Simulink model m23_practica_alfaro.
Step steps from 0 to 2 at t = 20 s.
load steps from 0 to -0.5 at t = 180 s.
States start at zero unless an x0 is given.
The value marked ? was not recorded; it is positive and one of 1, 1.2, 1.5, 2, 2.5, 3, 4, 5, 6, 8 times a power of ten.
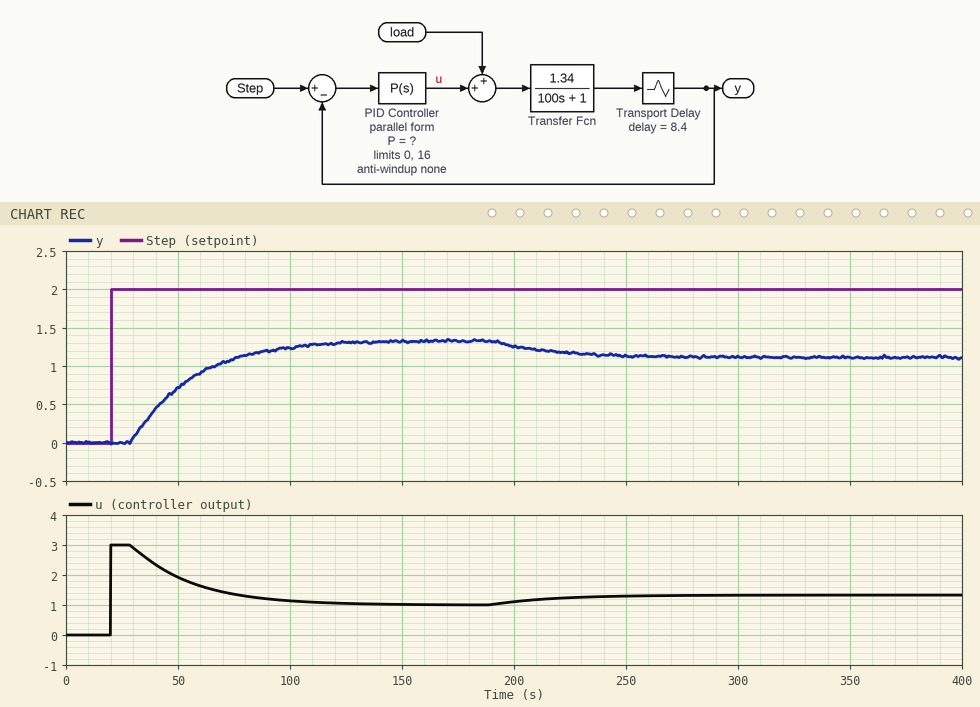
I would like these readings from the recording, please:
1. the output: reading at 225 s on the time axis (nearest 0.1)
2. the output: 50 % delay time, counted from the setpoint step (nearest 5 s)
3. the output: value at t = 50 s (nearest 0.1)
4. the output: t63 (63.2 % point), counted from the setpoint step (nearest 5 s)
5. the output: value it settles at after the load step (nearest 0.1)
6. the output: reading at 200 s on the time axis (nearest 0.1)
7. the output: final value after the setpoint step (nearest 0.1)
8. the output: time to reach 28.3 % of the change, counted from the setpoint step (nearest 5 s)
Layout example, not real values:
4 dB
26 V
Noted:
1.2
30 s
0.7
35 s
1.1
1.3
1.3
20 s
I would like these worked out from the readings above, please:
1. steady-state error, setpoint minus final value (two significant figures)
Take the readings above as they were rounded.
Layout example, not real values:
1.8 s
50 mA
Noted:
0.70
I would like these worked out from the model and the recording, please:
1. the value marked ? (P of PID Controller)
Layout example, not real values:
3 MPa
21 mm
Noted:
1.5
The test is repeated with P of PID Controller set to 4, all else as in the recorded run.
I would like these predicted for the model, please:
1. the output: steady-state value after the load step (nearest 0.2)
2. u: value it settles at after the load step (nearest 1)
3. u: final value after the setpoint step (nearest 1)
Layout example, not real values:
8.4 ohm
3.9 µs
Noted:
1.6
2
1
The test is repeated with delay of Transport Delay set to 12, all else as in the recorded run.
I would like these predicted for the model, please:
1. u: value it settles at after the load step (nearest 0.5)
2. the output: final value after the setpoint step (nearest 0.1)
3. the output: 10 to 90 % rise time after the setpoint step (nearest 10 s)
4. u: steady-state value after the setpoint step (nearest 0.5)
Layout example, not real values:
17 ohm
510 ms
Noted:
1.5
1.3
50 s
1.0
